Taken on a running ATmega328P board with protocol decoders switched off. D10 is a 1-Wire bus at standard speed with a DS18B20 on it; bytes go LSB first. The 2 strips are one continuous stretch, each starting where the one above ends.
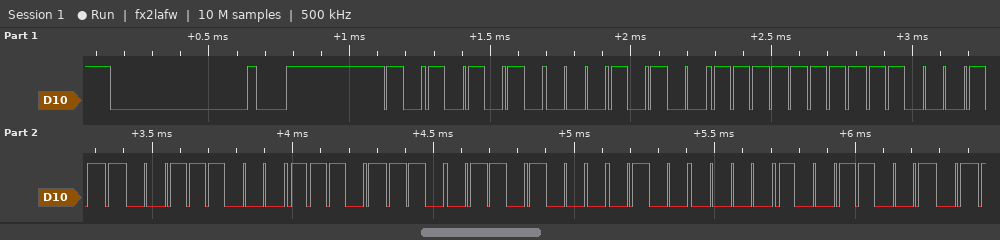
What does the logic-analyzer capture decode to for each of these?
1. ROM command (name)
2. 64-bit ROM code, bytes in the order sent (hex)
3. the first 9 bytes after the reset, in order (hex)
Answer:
Match ROM
28 FF E3 1C 77 16 02 99
55 28 FF E3 1C 77 16 02 99
